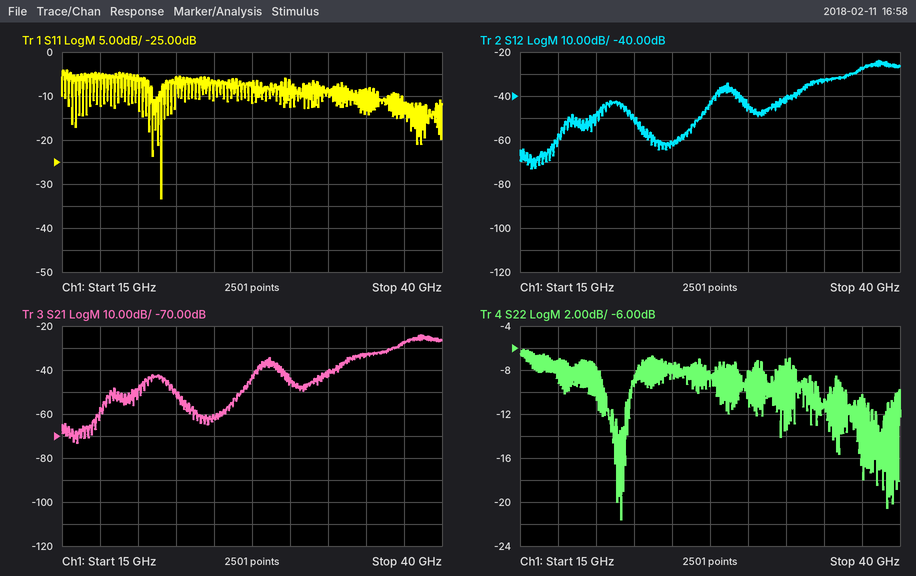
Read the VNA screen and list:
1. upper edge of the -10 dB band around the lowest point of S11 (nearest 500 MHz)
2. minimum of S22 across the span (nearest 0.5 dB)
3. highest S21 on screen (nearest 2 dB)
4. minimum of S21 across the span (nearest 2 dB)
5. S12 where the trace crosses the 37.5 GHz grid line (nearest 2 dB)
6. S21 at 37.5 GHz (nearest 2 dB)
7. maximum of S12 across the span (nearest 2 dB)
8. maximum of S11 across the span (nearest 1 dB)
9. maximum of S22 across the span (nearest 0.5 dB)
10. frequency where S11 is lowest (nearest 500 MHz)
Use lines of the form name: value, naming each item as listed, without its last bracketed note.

upper edge of the -10 dB band around the lowest point of S11: 21.5 GHz
minimum of S22 across the span: -21.5 dB
highest S21 on screen: -24 dB
minimum of S21 across the span: -74 dB
S12 where the trace crosses the 37.5 GHz grid line: -28 dB
S21 at 37.5 GHz: -28 dB
maximum of S12 across the span: -24 dB
maximum of S11 across the span: -4 dB
maximum of S22 across the span: -6.0 dB
frequency where S11 is lowest: 21.5 GHz
